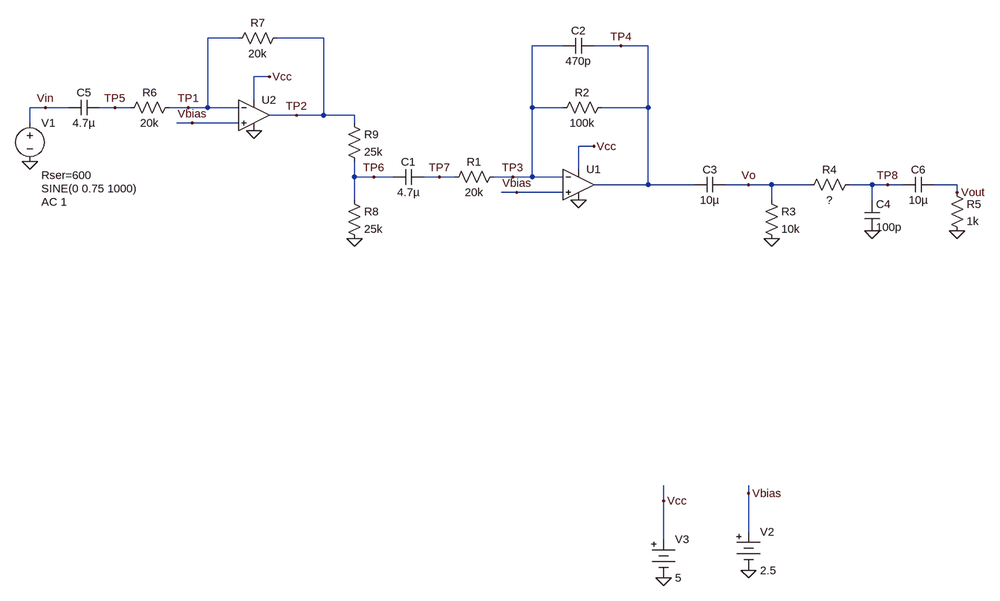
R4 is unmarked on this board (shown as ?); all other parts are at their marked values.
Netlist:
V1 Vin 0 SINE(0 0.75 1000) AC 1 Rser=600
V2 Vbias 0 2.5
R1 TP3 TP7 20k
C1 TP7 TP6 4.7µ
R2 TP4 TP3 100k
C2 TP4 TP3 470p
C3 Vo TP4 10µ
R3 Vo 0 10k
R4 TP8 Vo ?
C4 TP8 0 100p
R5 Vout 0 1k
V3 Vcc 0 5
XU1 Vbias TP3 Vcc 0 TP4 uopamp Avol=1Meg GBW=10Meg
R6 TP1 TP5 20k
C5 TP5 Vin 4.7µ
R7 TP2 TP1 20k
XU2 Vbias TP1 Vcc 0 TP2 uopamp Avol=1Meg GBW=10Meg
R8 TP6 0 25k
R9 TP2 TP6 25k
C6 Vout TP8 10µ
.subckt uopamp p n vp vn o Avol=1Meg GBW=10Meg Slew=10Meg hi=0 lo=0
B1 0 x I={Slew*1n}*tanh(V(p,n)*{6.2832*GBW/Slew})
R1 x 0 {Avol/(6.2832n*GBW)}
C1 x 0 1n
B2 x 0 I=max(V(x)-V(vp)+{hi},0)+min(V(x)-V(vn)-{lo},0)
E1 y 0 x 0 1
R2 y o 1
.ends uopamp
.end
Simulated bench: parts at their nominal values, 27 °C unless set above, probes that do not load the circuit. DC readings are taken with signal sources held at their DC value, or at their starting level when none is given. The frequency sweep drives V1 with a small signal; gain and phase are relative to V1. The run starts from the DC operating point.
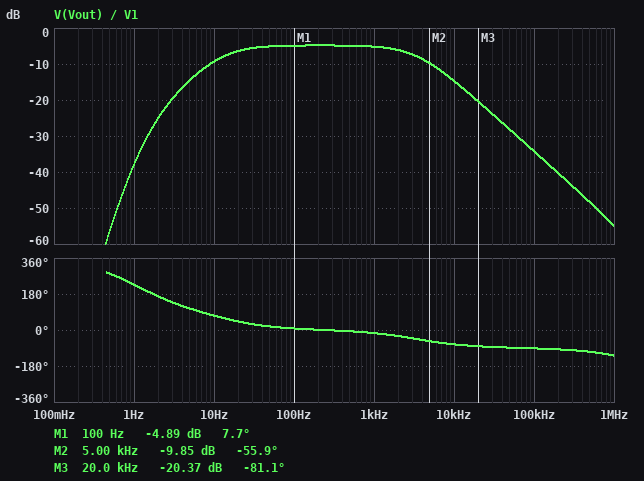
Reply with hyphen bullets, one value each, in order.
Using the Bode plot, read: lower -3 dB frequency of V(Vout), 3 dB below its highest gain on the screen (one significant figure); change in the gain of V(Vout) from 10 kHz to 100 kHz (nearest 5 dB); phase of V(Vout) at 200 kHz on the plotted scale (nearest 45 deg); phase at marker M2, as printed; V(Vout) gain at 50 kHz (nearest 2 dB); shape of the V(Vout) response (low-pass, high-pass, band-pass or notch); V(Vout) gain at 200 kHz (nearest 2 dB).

- 10 Hz
- -20 dB
- -90 deg
- -55.9 deg
- -28 dB
- band-pass
- -40 dB
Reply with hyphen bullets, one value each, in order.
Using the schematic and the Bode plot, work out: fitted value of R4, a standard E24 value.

- 1.6 kΩ
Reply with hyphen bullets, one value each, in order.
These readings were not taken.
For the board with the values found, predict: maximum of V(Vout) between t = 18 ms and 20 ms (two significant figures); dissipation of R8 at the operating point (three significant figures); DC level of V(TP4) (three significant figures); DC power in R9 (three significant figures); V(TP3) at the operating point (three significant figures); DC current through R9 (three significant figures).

- 410 mV
- 62.5 µW
- 2.50 V
- 62.5 µW
- 2.50 V
- 50.0 µA
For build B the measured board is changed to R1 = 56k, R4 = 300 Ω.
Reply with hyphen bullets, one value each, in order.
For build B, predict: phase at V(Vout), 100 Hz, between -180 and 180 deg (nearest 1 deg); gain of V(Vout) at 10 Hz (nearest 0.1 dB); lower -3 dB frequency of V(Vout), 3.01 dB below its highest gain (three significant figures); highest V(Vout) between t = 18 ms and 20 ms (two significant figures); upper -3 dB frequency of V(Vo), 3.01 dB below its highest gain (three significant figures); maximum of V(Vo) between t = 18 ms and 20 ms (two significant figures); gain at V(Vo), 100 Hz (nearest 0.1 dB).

- 14 deg
- -14.1 dB
- 25.1 Hz
- 390 mV
- 3.43 kHz
- 510 mV
- -3.2 dB
